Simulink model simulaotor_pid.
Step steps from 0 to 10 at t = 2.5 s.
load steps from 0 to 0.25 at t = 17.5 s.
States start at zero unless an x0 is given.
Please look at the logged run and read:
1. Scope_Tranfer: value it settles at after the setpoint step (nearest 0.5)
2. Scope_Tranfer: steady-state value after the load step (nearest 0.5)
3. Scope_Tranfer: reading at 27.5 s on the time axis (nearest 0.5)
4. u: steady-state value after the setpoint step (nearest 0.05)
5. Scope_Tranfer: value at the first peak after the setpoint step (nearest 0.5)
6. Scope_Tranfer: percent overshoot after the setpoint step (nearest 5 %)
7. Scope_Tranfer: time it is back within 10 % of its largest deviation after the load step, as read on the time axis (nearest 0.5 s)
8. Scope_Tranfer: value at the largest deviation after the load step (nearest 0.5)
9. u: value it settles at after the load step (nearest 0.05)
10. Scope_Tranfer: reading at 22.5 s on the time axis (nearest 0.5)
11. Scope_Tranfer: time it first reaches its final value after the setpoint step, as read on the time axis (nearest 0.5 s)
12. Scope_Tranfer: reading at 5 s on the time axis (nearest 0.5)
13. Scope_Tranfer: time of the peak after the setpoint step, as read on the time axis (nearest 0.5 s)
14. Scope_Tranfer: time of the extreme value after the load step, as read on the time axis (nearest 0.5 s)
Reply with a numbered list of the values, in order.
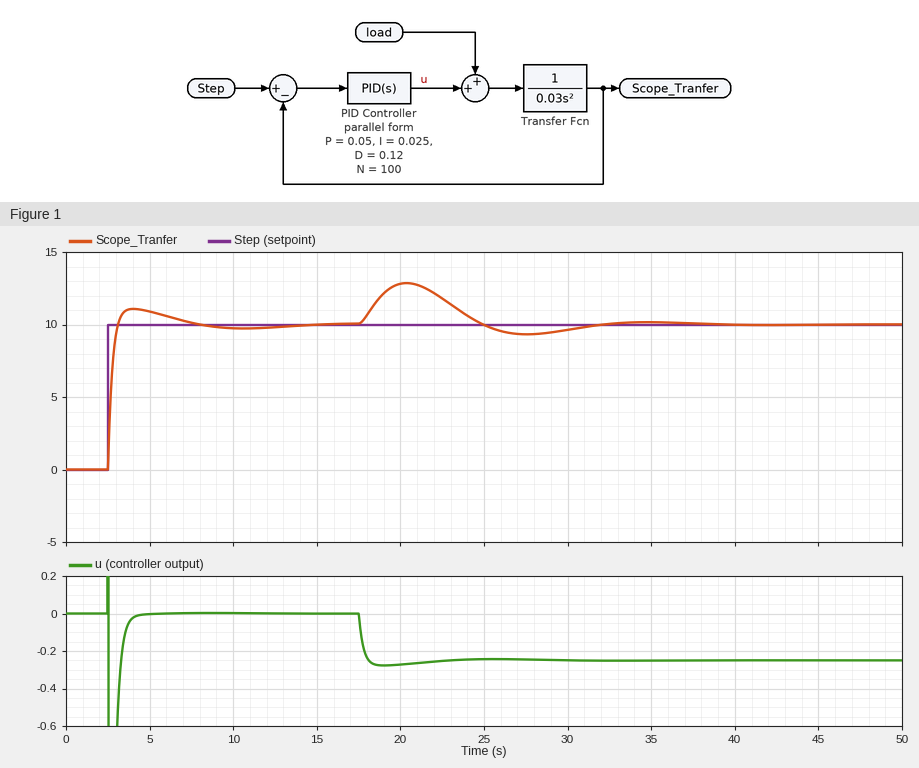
1. 10.0
2. 10.0
3. 9.5
4. 0.00
5. 11.0
6. 10 %
7. 30.5 s
8. 13.0
9. -0.25
10. 12.0
11. 3.0 s
12. 11.0
13. 4.0 s
14. 20.5 s
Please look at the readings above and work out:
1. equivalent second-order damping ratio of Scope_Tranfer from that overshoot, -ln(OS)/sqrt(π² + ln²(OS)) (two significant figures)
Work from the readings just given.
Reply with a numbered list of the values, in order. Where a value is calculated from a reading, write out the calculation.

1. ln(0.1) = -2.303; 2.303 / sqrt(9.870 + 5.302) = 0.59
